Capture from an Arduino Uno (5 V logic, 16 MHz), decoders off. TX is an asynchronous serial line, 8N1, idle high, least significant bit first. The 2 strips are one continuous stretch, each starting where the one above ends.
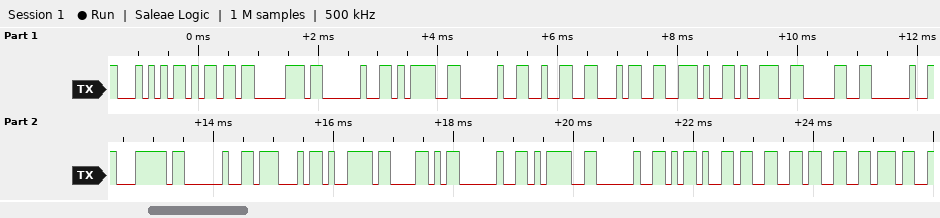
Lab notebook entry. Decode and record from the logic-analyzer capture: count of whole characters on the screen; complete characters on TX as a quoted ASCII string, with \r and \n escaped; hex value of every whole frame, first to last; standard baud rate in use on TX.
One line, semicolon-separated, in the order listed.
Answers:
24; "Tmp = 24.90 | GyX = -337"; 54 6D 70 20 3D 20 32 34 2E 39 30 20 7C 20 47 79 58 20 3D 20 2D 33 33 37; 9600 baud
